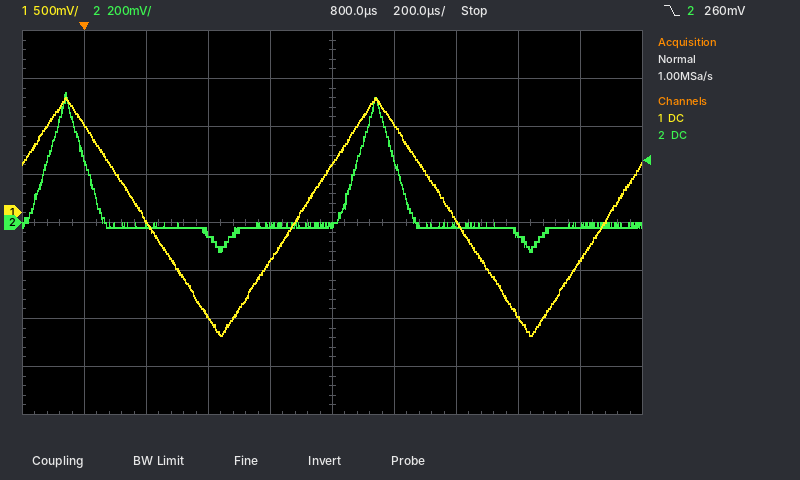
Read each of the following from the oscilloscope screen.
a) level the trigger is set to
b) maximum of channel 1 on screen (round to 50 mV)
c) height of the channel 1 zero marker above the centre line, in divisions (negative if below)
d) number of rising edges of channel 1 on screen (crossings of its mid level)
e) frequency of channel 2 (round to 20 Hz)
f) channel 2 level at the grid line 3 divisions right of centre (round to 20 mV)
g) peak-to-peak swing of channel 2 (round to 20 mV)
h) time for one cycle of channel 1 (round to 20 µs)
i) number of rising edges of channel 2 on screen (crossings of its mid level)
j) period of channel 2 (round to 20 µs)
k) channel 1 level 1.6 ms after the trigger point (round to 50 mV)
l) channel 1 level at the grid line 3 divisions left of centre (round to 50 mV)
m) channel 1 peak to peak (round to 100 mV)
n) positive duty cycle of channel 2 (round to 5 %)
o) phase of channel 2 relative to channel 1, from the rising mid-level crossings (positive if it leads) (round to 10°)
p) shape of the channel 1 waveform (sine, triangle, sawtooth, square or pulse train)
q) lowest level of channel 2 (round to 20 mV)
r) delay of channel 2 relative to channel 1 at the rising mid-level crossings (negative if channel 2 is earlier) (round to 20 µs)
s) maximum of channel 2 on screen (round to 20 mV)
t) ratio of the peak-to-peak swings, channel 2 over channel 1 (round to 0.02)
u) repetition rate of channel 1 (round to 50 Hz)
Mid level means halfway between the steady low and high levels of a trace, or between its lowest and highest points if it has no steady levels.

260 mV
1.20 V
+0.2 div
2
1.00 kHz
-40 mV
660 mV
1.00 ms
2
1.00 ms
-500 mV
-100 mV
2.50 V
15 %
-60°
triangle
-120 mV
+180 µs
540 mV
0.26
1.00 kHz
